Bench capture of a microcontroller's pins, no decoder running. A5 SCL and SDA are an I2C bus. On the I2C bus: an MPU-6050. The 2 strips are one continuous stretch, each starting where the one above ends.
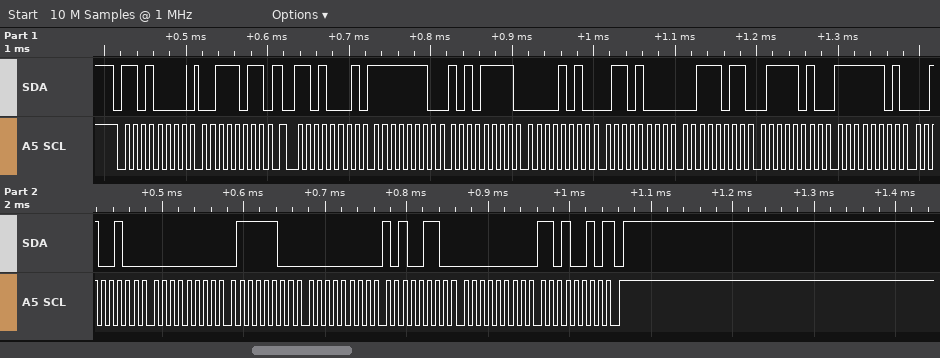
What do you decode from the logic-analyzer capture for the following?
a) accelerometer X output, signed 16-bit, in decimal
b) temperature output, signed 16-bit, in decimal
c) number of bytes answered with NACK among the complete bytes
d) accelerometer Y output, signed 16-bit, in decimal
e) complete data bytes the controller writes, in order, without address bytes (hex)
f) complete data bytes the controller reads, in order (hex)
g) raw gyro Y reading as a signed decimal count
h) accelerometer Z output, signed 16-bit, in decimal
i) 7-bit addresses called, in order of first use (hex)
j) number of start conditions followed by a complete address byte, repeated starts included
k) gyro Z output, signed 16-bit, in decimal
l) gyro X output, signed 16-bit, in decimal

-337
-732
1
2664
3B
FE AF 0A 68 3B 7A FD 24 00 7C 00 A6 00 D2
166
15226
0x68
2
210
124
